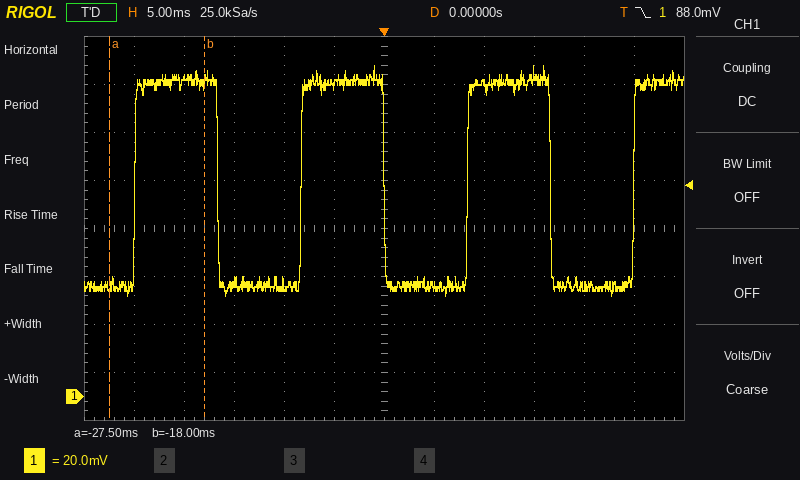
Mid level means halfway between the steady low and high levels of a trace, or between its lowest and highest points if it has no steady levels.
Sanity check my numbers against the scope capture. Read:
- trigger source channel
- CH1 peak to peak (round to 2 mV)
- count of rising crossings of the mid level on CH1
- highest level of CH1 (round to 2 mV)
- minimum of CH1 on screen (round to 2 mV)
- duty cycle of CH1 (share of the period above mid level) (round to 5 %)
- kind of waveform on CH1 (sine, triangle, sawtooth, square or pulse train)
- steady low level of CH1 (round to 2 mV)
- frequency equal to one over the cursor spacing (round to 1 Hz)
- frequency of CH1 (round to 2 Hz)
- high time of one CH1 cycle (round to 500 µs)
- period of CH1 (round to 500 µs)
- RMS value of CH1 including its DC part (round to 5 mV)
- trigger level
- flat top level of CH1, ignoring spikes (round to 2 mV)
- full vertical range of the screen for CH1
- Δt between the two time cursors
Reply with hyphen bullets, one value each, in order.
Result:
- CH1
- 96 mV
- 4
- 138 mV
- 42 mV
- 50 %
- square
- 46 mV
- 105 Hz
- 60 Hz
- 8.5 ms
- 16.5 ms
- 100 mV
- 88.0 mV
- 132 mV
- 160 mV
- 9.5 ms
